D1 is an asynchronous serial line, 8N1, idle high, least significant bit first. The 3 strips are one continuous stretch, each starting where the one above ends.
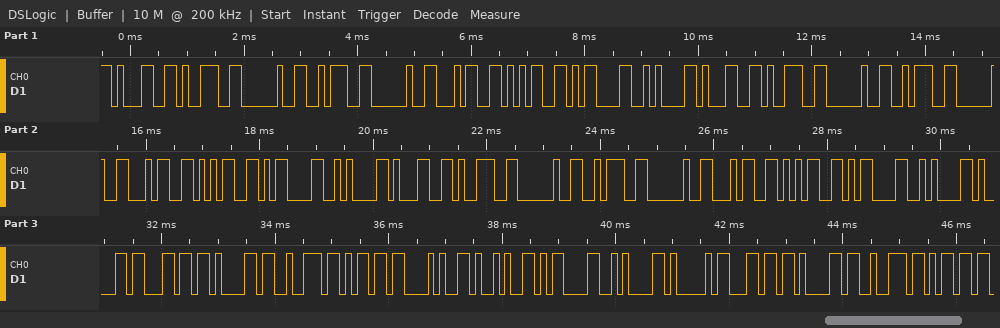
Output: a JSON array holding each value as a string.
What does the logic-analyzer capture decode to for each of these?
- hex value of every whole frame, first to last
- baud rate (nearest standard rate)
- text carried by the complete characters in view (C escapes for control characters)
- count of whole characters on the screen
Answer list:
["31 39 20 3A 20 34 35 0D 0A 31 39 20 3A 20 34 35 0D 0A 31 39 20 3A 20 34 35 0D 0A 61 6C 61 72 6D 28 29 0D 0A 41 6C 61 72 6D", "9600 baud", "\"19 : 45\\r\\n19 : 45\\r\\n19 : 45\\r\\nalarm()\\r\\nAlarm\"", "41"]
